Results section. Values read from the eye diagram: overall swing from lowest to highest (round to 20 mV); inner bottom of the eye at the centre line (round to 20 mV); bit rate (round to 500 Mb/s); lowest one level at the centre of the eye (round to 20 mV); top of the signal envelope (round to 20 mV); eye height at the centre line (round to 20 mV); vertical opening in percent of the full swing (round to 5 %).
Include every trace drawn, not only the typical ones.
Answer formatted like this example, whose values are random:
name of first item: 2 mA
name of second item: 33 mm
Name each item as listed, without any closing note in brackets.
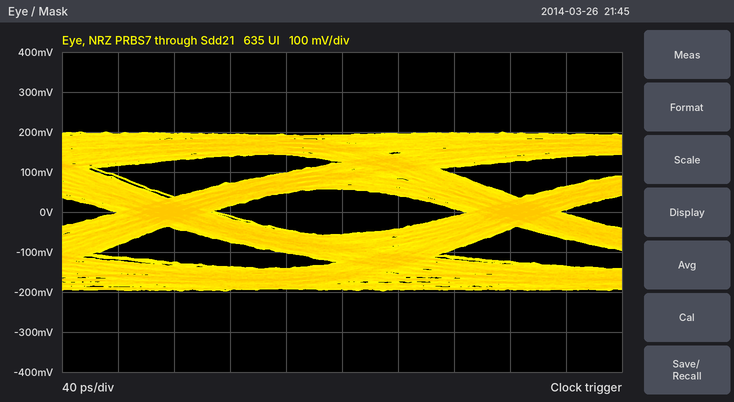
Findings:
overall swing from lowest to highest: 400 mV
inner bottom of the eye at the centre line: -60 mV
bit rate: 4.0 Gb/s
lowest one level at the centre of the eye: 60 mV
top of the signal envelope: 200 mV
eye height at the centre line: 120 mV
vertical opening in percent of the full swing: 30 %
